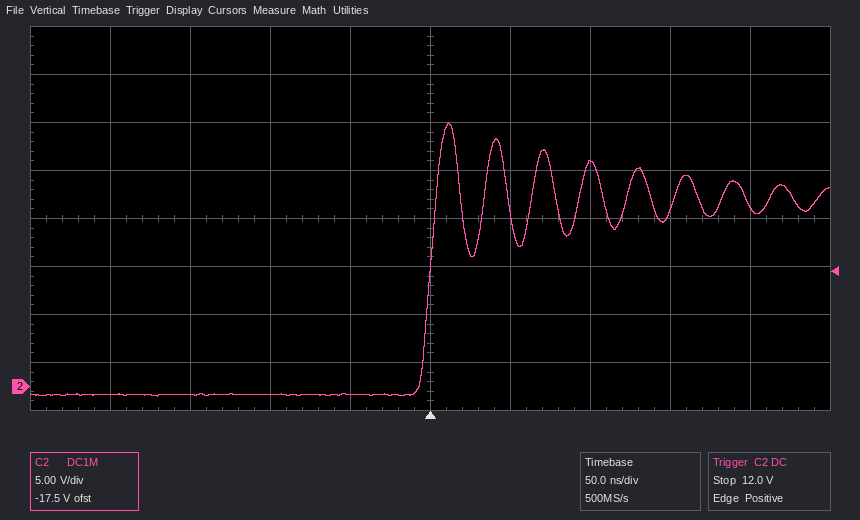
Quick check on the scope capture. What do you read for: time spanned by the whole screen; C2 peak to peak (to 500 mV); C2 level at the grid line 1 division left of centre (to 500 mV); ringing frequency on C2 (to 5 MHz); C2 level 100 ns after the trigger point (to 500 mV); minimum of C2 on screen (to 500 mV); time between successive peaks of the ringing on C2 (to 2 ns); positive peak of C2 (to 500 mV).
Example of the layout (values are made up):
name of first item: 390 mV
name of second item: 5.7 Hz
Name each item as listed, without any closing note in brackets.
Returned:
time spanned by the whole screen: 500 ns
C2 peak to peak: 28.5 V
C2 level at the grid line 1 division left of centre: -1.0 V
ringing frequency on C2: 35 MHz
C2 level 100 ns after the trigger point: 23.0 V
minimum of C2 on screen: -1.0 V
time between successive peaks of the ringing on C2: 30 ns
positive peak of C2: 27.5 V
